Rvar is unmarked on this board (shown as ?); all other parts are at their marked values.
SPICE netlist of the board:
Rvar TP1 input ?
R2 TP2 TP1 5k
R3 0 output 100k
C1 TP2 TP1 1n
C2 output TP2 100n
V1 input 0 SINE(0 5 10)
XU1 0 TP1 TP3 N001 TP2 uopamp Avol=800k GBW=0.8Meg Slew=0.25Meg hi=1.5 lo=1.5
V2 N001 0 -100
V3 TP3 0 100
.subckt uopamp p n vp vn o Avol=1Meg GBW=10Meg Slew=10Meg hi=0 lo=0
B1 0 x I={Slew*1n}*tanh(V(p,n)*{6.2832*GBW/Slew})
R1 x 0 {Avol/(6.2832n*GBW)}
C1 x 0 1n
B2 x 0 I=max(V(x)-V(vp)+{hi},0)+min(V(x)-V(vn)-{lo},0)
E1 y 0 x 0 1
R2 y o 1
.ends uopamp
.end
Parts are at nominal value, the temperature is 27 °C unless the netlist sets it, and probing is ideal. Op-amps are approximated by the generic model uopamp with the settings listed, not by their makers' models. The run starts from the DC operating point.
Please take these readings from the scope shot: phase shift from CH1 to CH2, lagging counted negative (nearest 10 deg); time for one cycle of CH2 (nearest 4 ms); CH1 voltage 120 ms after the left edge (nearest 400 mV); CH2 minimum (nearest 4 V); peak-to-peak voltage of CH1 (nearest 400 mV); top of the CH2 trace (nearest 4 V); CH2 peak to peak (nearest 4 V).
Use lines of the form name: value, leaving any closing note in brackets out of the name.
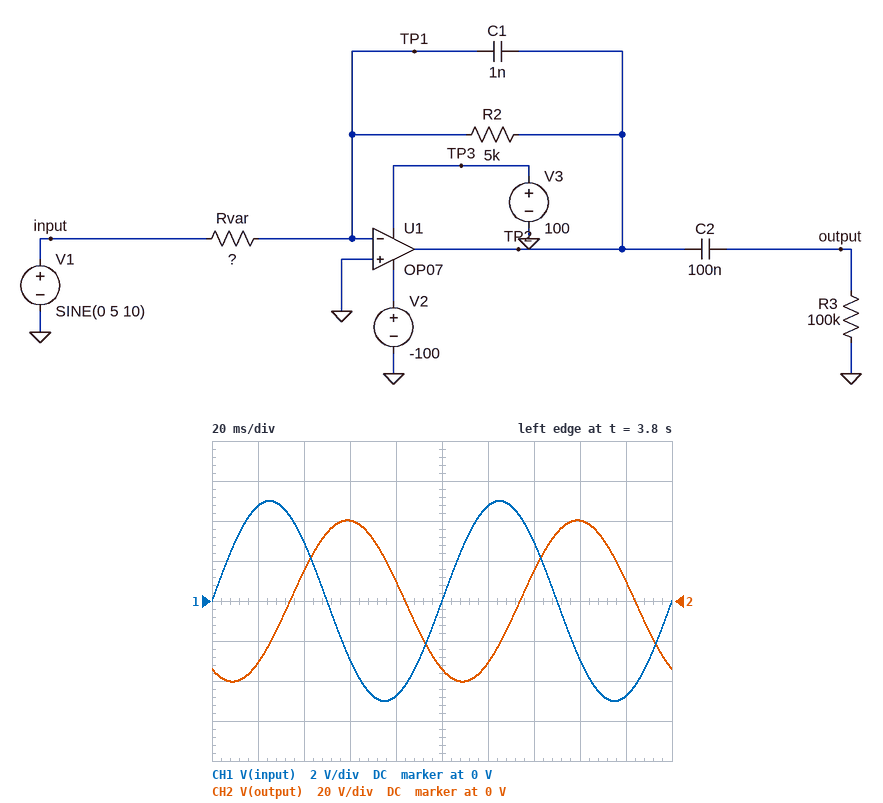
phase shift from CH1 to CH2, lagging counted negative: -120 deg
time for one cycle of CH2: 100 ms
CH1 voltage 120 ms after the left edge: 4.8 V
CH2 minimum: -40 V
peak-to-peak voltage of CH1: 10.0 V
top of the CH2 trace: 40 V
CH2 peak to peak: 80 V
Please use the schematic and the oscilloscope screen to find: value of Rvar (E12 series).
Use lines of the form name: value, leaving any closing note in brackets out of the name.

value of Rvar: 330 Ω
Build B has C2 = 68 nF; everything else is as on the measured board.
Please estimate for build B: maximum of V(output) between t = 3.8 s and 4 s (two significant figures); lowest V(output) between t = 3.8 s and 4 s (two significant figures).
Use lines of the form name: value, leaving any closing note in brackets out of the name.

maximum of V(output) between t = 3.8 s and 4 s: 30 V
lowest V(output) between t = 3.8 s and 4 s: -30 V
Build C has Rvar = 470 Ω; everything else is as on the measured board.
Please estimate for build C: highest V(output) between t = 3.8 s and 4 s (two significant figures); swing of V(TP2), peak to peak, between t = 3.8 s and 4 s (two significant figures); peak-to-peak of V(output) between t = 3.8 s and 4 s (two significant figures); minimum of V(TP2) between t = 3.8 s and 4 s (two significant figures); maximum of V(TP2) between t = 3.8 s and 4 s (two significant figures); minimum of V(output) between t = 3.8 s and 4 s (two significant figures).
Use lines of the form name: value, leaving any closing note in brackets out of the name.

highest V(output) between t = 3.8 s and 4 s: 28 V
swing of V(TP2), peak to peak, between t = 3.8 s and 4 s: 110 V
peak-to-peak of V(output) between t = 3.8 s and 4 s: 57 V
minimum of V(TP2) between t = 3.8 s and 4 s: -53 V
maximum of V(TP2) between t = 3.8 s and 4 s: 53 V
minimum of V(output) between t = 3.8 s and 4 s: -28 V
